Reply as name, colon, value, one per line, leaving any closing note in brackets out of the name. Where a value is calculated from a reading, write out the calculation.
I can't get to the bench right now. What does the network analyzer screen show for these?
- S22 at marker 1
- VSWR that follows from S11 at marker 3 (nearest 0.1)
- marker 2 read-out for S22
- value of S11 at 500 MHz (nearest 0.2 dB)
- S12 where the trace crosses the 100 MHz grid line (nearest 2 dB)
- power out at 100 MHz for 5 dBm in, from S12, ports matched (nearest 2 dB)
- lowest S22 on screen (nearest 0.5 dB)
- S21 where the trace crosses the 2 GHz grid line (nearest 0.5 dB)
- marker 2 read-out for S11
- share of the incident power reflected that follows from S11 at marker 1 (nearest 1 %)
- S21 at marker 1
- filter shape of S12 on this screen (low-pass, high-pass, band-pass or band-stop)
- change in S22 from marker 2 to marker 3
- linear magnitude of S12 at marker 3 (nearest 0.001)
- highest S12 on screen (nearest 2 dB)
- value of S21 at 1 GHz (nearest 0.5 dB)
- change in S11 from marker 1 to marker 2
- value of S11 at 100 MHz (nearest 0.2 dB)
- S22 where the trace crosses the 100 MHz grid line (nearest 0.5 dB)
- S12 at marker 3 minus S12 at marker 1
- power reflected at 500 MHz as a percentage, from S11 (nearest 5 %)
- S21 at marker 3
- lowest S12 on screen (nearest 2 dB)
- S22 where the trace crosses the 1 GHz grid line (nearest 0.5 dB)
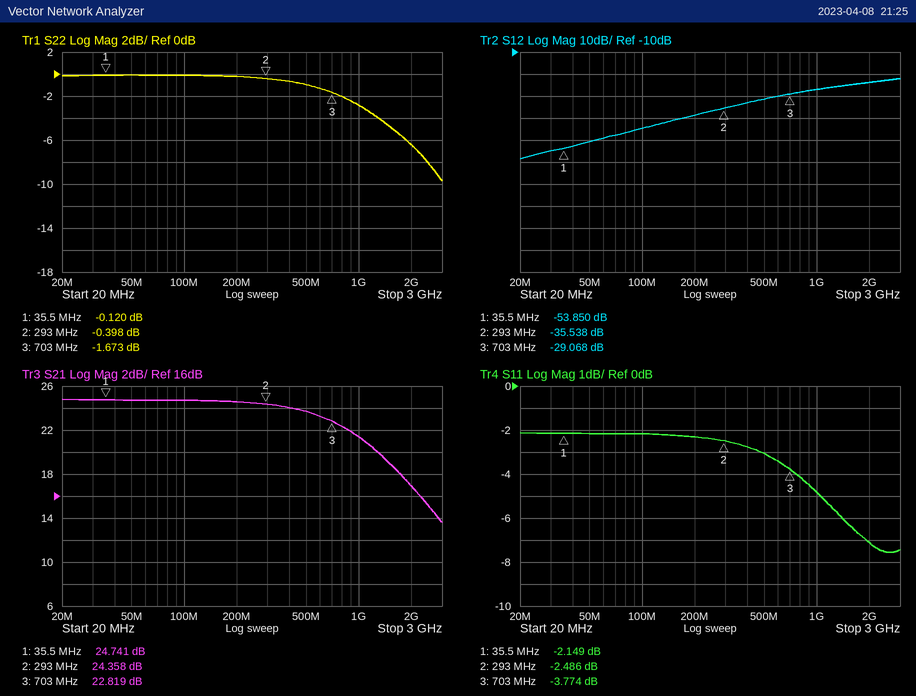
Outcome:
S22 at marker 1: -0.120 dB
VSWR that follows from S11 at marker 3: (1 + 0.6476)/(1 − 0.6476) ≈ 4.7
marker 2 read-out for S22: -0.398 dB
value of S11 at 500 MHz: -3.0 dB
S12 where the trace crosses the 100 MHz grid line: -44 dB
power out at 100 MHz for 5 dBm in, from S12, ports matched: 5 dBm + (-44 dB) = -40 dBm
lowest S22 on screen: -9.5 dB
S21 where the trace crosses the 2 GHz grid line: 17.0 dB
marker 2 read-out for S11: -2.486 dB
share of the incident power reflected that follows from S11 at marker 1: 10^(-2.149/10) ≈ 61 %
S21 at marker 1: 24.741 dB
filter shape of S12 on this screen: high-pass
change in S22 from marker 2 to marker 3: -1.673 − (-0.398) = -1.275 dB
linear magnitude of S12 at marker 3: 10^(-29.068/20) ≈ 0.035
highest S12 on screen: -22 dB
value of S21 at 1 GHz: 21.5 dB
change in S11 from marker 1 to marker 2: -2.486 − (-2.149) = -0.337 dB
value of S11 at 100 MHz: -2.2 dB
S22 where the trace crosses the 100 MHz grid line: 0.0 dB
S12 at marker 3 minus S12 at marker 1: -29.068 − (-53.85) = 24.782 dB
power reflected at 500 MHz as a percentage, from S11: 10^(-3/10) ≈ 50 %
S21 at marker 3: 22.819 dB
lowest S12 on screen: -58 dB
S22 where the trace crosses the 1 GHz grid line: -3.0 dB
